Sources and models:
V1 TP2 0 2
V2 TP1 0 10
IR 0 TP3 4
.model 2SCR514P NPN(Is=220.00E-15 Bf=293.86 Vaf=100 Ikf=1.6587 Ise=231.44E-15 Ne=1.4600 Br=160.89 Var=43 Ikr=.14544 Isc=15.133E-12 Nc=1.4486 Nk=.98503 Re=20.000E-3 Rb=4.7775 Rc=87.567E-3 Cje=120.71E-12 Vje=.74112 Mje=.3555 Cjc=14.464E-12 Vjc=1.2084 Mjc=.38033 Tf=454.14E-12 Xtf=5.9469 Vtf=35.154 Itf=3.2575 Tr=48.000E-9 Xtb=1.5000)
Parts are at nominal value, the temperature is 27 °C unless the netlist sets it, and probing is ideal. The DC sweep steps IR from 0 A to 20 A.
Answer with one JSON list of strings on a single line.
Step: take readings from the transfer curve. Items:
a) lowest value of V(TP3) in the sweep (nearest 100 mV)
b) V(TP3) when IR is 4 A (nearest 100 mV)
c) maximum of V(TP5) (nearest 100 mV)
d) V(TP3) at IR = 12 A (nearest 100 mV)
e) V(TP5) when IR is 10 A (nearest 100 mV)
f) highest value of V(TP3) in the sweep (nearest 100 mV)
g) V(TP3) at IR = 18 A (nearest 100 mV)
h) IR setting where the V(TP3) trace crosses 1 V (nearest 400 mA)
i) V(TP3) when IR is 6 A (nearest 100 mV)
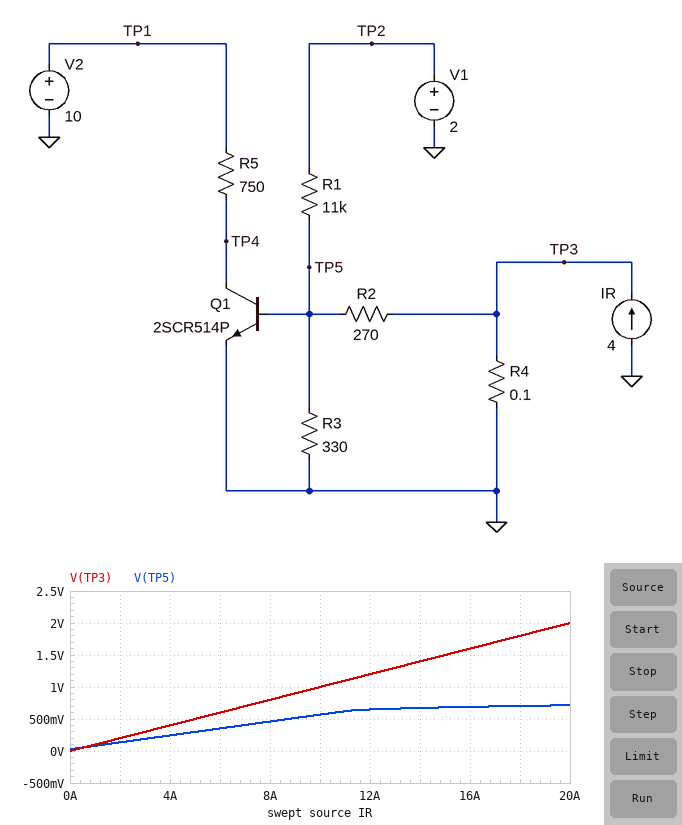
["0 V", "400 mV", "700 mV", "1.2 V", "600 mV", "2.0 V", "1.8 V", "10.0 A", "600 mV"]
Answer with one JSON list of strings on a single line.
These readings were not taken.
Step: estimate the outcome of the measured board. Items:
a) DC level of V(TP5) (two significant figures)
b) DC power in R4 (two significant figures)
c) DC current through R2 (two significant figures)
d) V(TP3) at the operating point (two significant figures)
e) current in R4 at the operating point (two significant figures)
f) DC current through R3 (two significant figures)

["240 mV", "1.6 W", "580 µA", "400 mV", "4.0 A", "740 µA"]
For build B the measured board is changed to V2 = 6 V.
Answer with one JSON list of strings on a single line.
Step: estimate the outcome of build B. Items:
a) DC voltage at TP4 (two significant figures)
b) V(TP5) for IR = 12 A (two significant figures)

["6.0 V", "640 mV"]
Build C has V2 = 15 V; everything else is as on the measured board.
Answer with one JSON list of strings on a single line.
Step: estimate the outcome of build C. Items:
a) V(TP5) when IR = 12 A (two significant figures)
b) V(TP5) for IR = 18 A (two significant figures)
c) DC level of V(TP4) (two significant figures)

["660 mV", "710 mV", "15 V"]
